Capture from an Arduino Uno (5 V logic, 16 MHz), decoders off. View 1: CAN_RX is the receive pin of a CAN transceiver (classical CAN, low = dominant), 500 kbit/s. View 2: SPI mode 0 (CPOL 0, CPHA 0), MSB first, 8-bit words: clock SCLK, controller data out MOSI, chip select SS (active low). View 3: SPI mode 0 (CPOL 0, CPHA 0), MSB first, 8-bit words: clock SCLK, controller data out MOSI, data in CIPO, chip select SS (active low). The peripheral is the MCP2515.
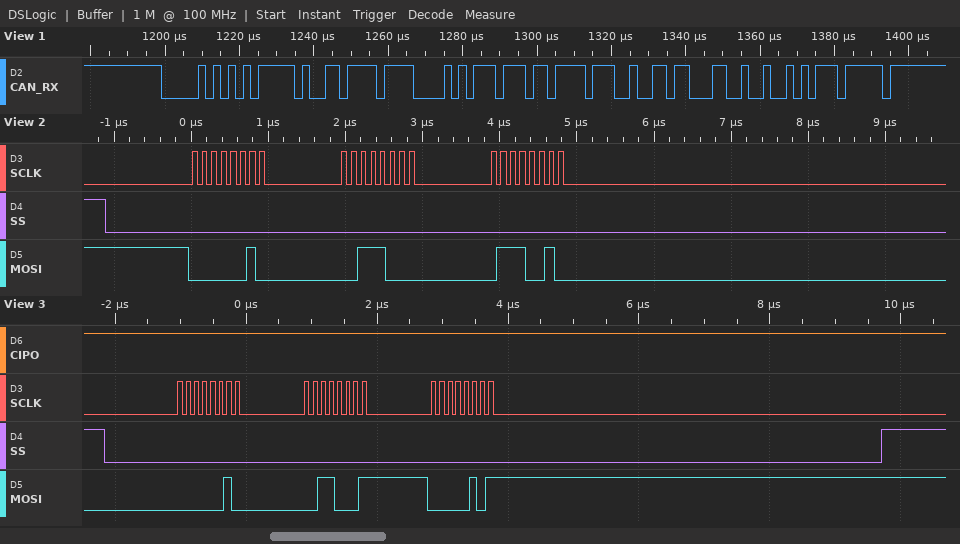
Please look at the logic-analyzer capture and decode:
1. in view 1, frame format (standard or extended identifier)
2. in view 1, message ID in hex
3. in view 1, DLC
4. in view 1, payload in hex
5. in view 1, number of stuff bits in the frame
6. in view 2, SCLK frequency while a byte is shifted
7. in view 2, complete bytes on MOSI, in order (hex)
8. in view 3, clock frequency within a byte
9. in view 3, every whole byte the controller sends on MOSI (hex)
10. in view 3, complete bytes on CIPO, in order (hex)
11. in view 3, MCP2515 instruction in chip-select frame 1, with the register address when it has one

extended
0x00ABCDEF
5
77 6F 72 6C 64
2
8 MHz
02 38 72
8 MHz
02 31 05
FF FF FF
WRITE 0x31
